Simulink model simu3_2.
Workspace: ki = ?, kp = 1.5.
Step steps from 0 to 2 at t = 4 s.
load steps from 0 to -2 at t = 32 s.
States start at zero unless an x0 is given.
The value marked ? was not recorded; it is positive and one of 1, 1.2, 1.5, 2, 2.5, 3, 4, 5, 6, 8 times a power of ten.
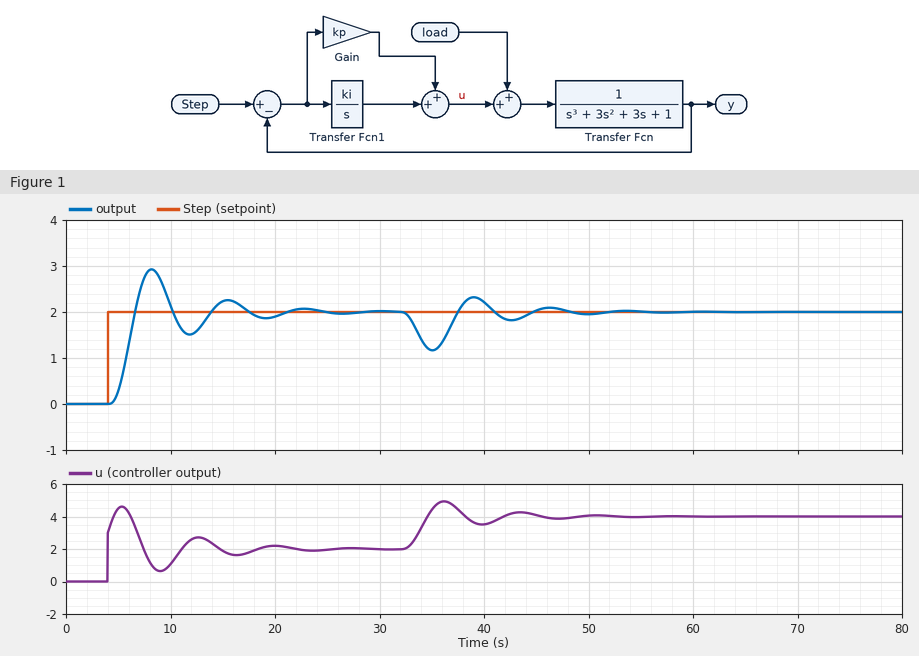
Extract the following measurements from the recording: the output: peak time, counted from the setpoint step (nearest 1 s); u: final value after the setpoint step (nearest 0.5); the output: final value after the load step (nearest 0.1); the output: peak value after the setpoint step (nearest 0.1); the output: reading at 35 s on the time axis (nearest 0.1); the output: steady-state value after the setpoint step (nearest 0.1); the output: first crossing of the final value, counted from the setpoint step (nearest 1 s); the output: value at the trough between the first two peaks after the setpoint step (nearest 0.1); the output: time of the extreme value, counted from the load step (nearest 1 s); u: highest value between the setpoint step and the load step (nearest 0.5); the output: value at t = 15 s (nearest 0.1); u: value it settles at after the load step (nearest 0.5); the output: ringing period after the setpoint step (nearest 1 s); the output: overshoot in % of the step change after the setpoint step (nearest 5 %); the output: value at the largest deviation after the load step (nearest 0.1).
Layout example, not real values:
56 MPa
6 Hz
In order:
4 s
2.0
2.0
2.9
1.2
2.0
3 s
1.5
3 s
4.5
2.2
4.0
7 s
45 %
1.2
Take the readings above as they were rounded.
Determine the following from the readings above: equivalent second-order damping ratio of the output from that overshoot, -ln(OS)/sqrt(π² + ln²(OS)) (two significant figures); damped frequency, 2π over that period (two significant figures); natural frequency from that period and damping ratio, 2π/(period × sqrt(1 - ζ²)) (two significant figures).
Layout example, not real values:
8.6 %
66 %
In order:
0.25
0.90 rad/s
0.93 rad/s
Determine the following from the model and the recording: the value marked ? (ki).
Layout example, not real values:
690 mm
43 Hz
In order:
1
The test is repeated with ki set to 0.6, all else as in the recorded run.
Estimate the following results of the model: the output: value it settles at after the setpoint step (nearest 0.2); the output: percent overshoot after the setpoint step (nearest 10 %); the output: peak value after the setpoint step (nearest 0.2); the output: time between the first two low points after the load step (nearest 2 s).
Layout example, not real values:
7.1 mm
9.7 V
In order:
2.0
20 %
2.4
8 s
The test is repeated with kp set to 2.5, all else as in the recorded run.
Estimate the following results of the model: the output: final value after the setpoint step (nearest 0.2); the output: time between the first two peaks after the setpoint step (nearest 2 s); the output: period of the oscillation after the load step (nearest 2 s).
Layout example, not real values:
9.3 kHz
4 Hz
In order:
2.0
6 s
6 s
